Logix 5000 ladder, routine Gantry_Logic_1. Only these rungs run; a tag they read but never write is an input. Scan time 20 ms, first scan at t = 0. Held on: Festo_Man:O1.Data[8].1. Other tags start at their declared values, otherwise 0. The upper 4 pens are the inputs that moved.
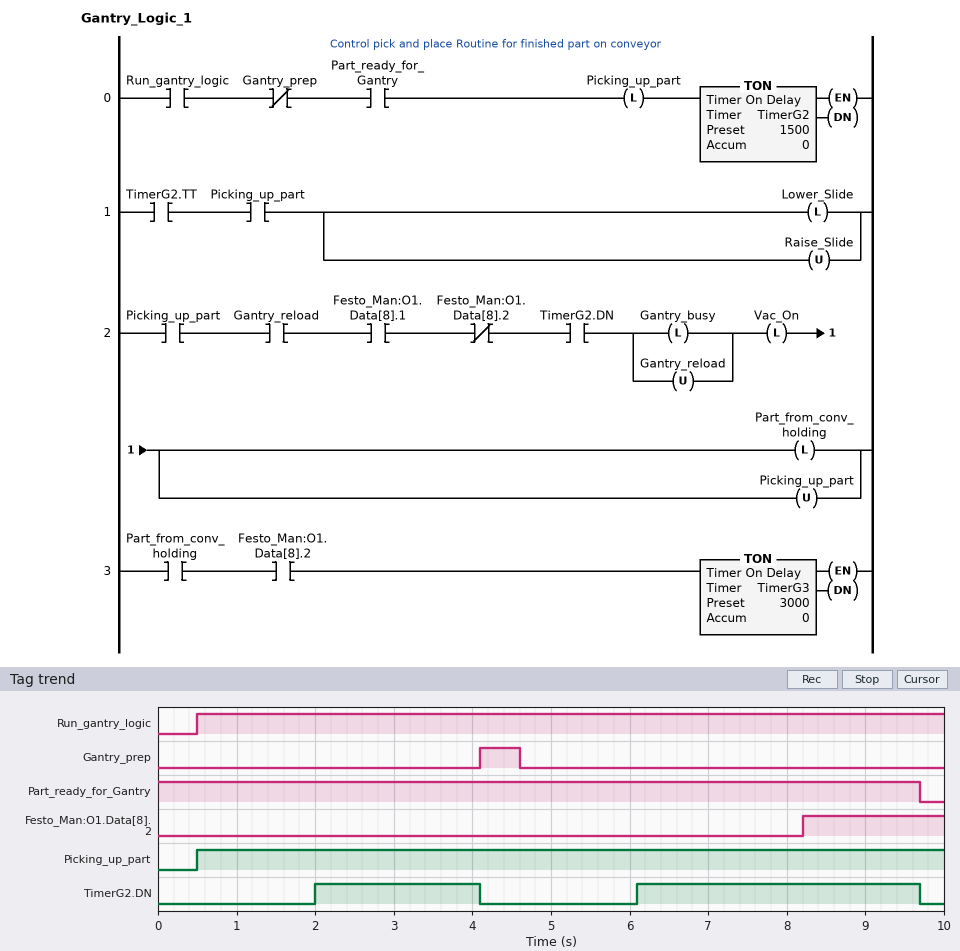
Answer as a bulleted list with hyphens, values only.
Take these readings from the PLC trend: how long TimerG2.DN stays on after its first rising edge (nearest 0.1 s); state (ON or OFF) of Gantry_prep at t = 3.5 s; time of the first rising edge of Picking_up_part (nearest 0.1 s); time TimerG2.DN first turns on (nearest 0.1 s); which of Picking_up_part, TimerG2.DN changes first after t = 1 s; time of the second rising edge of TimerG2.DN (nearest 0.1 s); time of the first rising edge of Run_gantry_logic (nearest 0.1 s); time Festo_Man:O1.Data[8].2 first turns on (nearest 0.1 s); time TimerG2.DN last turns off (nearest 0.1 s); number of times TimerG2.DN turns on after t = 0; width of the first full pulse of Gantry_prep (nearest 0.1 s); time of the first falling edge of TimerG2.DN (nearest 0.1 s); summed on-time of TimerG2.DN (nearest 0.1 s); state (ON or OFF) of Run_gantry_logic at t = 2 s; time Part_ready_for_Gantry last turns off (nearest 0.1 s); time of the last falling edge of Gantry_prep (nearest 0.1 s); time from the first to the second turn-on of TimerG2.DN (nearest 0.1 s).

- 2.1 s
- OFF
- 0.5 s
- 2.0 s
- TimerG2.DN
- 6.1 s
- 0.5 s
- 8.2 s
- 9.7 s
- 2
- 0.5 s
- 4.1 s
- 5.7 s
- ON
- 9.7 s
- 4.6 s
- 4.1 s
